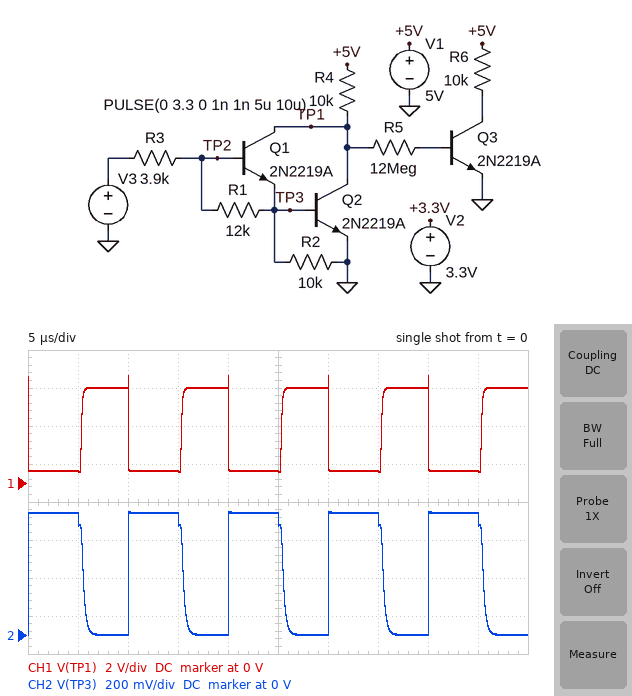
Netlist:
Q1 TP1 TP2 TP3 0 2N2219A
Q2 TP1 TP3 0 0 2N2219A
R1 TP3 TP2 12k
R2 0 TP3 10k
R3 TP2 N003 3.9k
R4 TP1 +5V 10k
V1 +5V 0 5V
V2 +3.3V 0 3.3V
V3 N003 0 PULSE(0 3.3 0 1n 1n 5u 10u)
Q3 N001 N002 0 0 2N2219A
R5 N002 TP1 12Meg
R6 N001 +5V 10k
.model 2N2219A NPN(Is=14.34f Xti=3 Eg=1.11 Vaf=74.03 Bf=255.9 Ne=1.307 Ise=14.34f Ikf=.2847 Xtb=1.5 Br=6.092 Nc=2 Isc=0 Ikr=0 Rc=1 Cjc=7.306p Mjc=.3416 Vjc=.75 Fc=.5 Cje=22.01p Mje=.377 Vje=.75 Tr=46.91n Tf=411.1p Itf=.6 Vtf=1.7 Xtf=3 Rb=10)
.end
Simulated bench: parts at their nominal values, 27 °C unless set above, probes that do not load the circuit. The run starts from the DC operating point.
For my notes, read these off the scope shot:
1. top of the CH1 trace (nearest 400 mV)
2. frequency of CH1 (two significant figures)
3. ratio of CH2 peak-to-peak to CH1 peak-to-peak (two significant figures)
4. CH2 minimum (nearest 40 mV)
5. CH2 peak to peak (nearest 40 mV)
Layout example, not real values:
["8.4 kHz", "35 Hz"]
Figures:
["5.6 V", "100 kHz", "0.13", "0 V", "640 mV"]
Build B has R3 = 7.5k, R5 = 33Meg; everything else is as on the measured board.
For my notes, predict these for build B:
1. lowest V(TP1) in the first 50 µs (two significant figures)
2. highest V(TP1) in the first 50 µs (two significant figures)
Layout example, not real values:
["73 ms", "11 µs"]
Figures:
["610 mV", "5.5 V"]
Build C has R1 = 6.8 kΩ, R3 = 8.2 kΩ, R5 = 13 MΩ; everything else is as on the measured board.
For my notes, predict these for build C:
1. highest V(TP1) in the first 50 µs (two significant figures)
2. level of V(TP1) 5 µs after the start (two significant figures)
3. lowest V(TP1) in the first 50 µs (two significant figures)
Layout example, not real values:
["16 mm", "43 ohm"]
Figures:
["5.5 V", "630 mV", "610 mV"]
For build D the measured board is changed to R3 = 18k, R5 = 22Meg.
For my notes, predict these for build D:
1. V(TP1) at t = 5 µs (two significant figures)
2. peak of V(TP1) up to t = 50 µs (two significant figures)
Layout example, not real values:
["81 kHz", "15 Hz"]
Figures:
["630 mV", "5.3 V"]
